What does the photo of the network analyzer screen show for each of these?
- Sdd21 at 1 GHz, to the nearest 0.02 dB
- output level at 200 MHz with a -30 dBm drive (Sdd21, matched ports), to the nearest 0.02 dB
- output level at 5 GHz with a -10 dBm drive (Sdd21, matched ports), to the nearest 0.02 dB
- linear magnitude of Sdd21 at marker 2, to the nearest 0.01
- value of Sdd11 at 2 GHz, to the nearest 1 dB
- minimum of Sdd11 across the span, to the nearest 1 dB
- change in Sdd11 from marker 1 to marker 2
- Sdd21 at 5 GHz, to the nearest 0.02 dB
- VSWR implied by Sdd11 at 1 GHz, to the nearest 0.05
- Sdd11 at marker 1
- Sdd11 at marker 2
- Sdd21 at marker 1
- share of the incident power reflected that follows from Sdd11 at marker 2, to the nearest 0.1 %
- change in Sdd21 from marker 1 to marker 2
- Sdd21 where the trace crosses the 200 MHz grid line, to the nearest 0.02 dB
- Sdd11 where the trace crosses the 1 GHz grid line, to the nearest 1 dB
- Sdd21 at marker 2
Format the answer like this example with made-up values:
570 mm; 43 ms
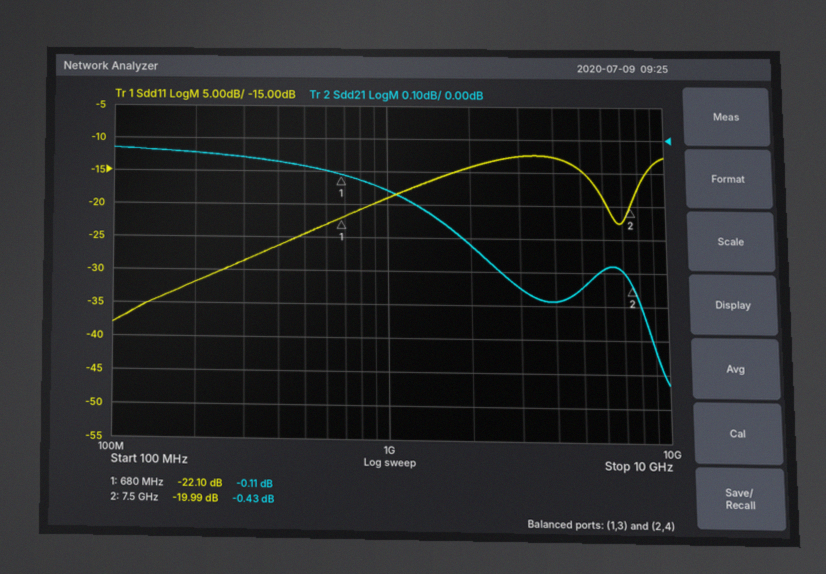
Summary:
-0.16 dB; -30.04 dBm; -10.44 dBm; 0.95; -14 dB; -38 dB; 2.11 dB; -0.44 dB; 1.25; -22.10 dB; -19.99 dB; -0.11 dB; 1.0 %; -0.32 dB; -0.04 dB; -19 dB; -0.43 dB
